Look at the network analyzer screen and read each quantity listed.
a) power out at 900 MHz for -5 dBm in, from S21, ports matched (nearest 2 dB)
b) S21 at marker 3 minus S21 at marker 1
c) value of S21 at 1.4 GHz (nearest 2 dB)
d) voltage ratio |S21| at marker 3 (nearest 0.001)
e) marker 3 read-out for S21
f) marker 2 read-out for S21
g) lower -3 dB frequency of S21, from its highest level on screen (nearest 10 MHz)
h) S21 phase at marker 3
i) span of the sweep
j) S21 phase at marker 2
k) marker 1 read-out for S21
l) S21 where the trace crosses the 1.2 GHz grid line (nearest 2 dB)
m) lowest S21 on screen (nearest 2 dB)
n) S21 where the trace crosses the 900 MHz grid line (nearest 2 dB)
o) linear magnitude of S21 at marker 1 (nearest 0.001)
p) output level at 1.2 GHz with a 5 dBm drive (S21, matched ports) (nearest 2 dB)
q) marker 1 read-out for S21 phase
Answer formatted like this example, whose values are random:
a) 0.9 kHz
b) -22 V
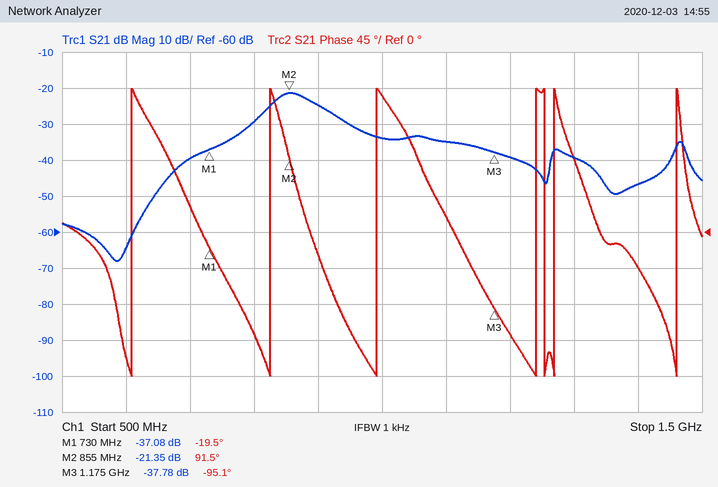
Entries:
a) -30 dBm
b) -0.70 dB
c) -46 dB
d) 0.013
e) -37.78 dB
f) -21.35 dB
g) 830 MHz
h) -95.1°
i) 1 GHz
j) 91.5°
k) -37.08 dB
l) -40 dB
m) -68 dB
n) -24 dB
o) 0.014
p) -34 dBm
q) -19.5°
